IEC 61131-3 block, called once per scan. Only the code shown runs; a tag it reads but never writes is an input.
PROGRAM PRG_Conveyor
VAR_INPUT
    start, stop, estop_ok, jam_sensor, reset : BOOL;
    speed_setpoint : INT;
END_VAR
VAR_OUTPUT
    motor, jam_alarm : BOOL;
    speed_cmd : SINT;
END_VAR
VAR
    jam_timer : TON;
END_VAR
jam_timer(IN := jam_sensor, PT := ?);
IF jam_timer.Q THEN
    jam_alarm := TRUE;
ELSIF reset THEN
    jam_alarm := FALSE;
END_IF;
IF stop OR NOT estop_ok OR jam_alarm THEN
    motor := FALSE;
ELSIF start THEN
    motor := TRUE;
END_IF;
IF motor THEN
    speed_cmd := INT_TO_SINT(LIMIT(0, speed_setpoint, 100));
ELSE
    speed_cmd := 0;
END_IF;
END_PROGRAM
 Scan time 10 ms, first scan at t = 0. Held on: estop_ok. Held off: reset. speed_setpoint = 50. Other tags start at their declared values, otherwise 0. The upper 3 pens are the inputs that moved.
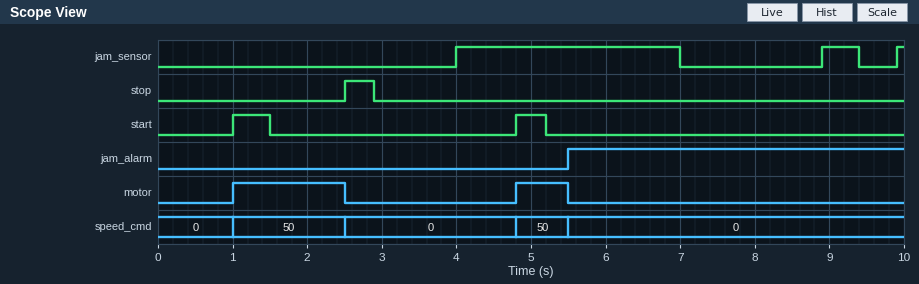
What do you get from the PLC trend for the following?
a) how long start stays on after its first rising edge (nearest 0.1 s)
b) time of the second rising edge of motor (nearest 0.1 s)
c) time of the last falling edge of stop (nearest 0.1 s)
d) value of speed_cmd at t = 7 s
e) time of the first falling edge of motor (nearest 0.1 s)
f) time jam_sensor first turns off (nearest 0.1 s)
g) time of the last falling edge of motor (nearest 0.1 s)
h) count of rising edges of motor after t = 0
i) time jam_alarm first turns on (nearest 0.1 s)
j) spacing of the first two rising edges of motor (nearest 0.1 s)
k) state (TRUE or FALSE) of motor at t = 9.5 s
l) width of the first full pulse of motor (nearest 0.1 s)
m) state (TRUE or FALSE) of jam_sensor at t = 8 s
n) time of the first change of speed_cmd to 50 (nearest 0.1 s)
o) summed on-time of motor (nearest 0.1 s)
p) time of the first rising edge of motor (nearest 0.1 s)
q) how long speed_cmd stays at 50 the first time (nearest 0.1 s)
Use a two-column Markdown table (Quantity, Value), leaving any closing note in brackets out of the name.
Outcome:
| Quantity | Value |
|---|---|
| how long start stays on after its first rising edge | 0.5 s |
| time of the second rising edge of motor | 4.8 s |
| time of the last falling edge of stop | 2.9 s |
| value of speed_cmd at t = 7 s | 0 |
| time of the first falling edge of motor | 2.5 s |
| time jam_sensor first turns off | 7.0 s |
| time of the last falling edge of motor | 5.5 s |
| count of rising edges of motor after t = 0 | 2 |
| time jam_alarm first turns on | 5.5 s |
| spacing of the first two rising edges of motor | 3.8 s |
| state (TRUE or FALSE) of motor at t = 9.5 s | FALSE |
| width of the first full pulse of motor | 1.5 s |
| state (TRUE or FALSE) of jam_sensor at t = 8 s | FALSE |
| time of the first change of speed_cmd to 50 | 1.0 s |
| summed on-time of motor | 2.2 s |
| time of the first rising edge of motor | 1.0 s |
| how long speed_cmd stays at 50 the first time | 1.5 s |
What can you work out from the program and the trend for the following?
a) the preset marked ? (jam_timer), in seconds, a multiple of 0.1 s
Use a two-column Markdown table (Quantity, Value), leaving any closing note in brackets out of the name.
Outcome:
| Quantity | Value |
|---|---|
| the preset marked ? (jam_timer), in seconds, a multiple of 0.1 s | 1.5 s |
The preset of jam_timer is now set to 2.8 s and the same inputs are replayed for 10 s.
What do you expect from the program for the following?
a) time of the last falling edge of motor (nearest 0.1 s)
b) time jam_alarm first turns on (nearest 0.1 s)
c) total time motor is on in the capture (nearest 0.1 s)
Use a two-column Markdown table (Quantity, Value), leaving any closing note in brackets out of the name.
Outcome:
| Quantity | Value |
|---|---|
| time of the last falling edge of motor | 6.8 s |
| time jam_alarm first turns on | 6.8 s |
| total time motor is on in the capture | 3.5 s |
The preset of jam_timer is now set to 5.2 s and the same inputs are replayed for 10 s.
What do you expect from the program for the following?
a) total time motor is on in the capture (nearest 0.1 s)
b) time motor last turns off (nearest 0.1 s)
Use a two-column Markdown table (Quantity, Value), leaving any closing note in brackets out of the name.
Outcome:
| Quantity | Value |
|---|---|
| total time motor is on in the capture | 6.7 s |
| time motor last turns off | 2.5 s |
